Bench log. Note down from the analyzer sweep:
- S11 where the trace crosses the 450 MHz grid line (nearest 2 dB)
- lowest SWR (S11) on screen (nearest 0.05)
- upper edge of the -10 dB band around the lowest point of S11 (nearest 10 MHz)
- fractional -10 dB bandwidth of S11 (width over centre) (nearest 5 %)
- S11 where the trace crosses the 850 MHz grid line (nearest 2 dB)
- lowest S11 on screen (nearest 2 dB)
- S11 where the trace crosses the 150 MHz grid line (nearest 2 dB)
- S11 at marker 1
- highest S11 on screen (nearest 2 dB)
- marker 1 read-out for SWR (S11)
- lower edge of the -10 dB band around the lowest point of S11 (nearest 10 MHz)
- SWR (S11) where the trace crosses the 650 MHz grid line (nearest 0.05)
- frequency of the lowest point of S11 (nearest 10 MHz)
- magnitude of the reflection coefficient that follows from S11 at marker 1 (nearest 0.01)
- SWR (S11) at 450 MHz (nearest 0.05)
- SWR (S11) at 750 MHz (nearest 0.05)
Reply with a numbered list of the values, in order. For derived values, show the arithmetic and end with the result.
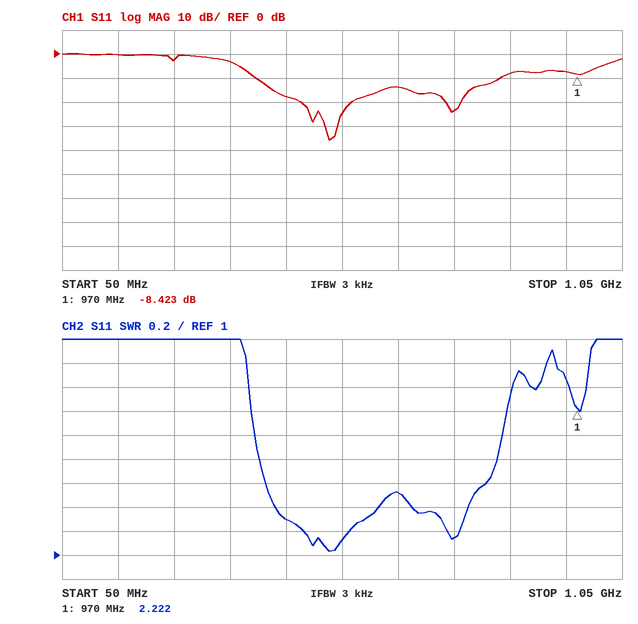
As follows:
1. -18 dB
2. 1.05
3. 830 MHz
4. 430 MHz / 615 MHz ≈ 70 %
5. -8 dB
6. -36 dB
7. 0 dB
8. -8.423 dB
9. 0 dB
10. 2.222
11. 400 MHz
12. 1.50
13. 530 MHz
14. 10^(-8.423/20) ≈ 0.38
15. 1.30
16. 1.15
